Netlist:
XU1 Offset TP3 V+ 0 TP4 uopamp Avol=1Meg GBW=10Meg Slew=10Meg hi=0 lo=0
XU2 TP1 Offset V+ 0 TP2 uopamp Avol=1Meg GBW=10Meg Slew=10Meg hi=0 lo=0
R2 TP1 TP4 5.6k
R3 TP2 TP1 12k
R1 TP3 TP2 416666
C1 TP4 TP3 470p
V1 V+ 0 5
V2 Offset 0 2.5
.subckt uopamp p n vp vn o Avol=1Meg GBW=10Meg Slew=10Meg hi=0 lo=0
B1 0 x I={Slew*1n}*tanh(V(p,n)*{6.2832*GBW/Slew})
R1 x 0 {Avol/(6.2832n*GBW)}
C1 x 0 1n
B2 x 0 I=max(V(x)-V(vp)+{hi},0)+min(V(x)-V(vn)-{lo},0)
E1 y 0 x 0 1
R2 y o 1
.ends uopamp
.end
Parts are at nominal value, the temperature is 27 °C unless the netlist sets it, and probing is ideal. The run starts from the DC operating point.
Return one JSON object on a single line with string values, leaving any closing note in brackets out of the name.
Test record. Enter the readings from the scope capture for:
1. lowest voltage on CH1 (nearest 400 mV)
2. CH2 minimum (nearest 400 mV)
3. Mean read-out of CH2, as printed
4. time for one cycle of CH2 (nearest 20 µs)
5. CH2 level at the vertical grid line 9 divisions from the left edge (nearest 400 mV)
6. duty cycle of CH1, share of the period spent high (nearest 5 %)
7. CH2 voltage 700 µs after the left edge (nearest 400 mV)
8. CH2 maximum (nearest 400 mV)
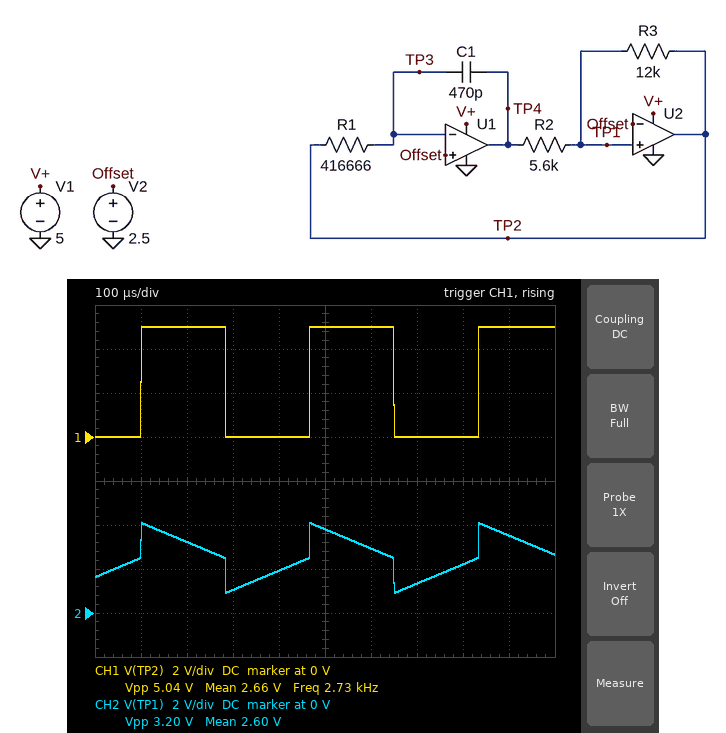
{"lowest voltage on CH1": "0 V", "CH2 minimum": "800 mV", "Mean read-out of CH2, as printed": "2.60 V", "time for one cycle of CH2": "360 µs", "CH2 level at the vertical grid line 9 divisions from the left edge": "3.6 V", "duty cycle of CH1, share of the period spent high": "50 %", "CH2 voltage 700 µs after the left edge": "1.2 V", "CH2 maximum": "4.0 V"}
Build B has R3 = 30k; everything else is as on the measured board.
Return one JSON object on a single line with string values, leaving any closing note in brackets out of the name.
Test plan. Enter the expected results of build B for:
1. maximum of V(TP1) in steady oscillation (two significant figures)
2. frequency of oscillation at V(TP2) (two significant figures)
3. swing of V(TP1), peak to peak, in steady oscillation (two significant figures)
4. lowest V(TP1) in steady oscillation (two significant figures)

{"maximum of V(TP1) in steady oscillation": "3.3 V", "frequency of oscillation at V(TP2)": "6.7 kHz", "swing of V(TP1), peak to peak, in steady oscillation": "1.6 V", "lowest V(TP1) in steady oscillation": "1.7 V"}
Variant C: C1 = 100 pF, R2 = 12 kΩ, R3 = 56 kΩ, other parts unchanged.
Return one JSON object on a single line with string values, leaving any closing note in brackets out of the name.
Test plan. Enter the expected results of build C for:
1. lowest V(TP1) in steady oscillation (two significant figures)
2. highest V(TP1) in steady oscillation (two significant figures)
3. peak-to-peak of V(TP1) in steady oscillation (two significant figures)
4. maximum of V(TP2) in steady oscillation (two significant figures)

{"lowest V(TP1) in steady oscillation": "1.6 V", "highest V(TP1) in steady oscillation": "3.4 V", "peak-to-peak of V(TP1) in steady oscillation": "1.8 V", "maximum of V(TP2) in steady oscillation": "5.0 V"}
